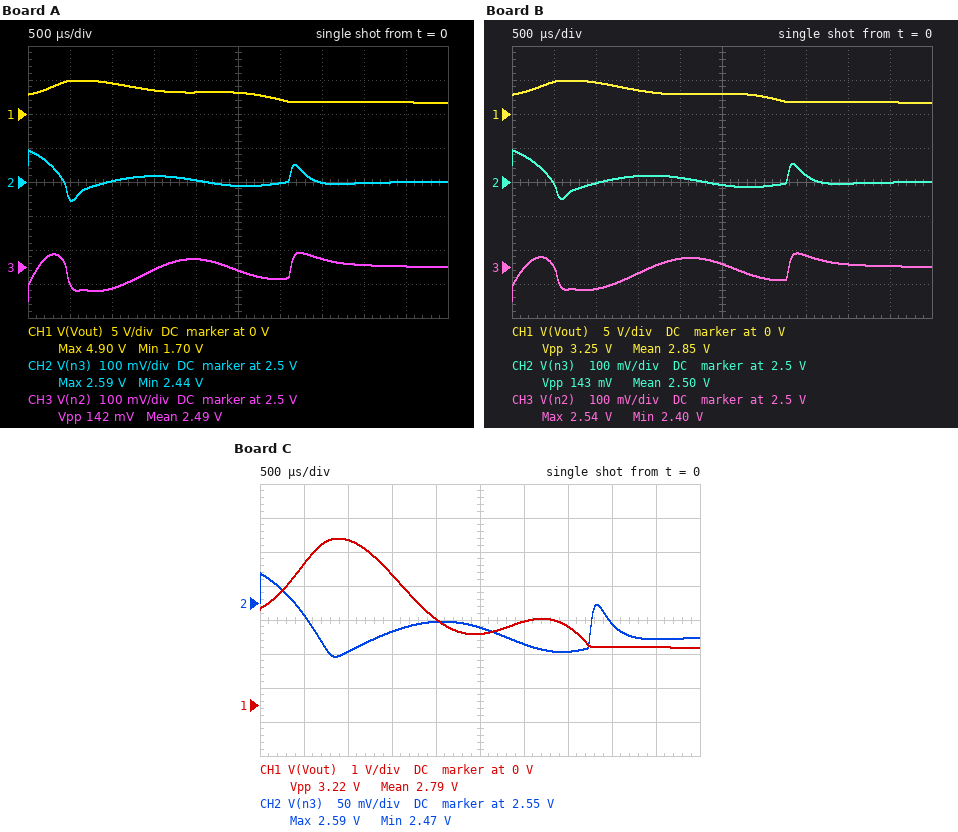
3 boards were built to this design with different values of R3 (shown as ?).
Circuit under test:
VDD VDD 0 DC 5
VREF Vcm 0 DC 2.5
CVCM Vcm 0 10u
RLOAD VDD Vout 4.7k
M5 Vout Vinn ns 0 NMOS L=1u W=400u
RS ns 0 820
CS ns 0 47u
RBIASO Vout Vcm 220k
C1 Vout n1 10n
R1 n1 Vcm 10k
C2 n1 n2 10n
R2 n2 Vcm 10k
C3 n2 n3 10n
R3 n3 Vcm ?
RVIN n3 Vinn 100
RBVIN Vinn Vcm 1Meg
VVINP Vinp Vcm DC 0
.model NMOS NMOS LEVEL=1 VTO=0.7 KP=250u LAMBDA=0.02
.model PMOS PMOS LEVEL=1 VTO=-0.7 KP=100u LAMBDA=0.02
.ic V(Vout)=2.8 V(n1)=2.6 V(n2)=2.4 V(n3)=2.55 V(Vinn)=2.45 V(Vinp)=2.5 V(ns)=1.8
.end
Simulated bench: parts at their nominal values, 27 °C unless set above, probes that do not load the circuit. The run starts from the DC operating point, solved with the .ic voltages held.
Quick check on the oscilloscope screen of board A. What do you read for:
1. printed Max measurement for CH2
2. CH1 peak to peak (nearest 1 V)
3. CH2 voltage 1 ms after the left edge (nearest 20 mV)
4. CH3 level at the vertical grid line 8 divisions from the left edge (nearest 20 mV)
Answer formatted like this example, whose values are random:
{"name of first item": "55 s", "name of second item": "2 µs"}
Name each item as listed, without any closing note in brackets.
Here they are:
{"printed Max measurement for CH2": "2.59 V", "CH1 peak to peak": "3 V", "CH2 voltage 1 ms after the left edge": "2.50 V", "CH3 level at the vertical grid line 8 divisions from the left edge": "2.50 V"}
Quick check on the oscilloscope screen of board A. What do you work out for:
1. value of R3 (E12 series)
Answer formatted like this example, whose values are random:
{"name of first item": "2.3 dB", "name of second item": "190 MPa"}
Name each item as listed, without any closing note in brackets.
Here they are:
{"value of R3": "15 kΩ"}
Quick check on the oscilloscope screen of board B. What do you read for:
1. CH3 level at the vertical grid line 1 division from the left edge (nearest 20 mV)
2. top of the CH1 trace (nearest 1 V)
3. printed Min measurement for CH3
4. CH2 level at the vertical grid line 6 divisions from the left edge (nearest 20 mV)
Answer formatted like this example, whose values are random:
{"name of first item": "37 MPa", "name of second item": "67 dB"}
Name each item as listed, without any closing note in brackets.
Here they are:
{"CH3 level at the vertical grid line 1 division from the left edge": "2.50 V", "top of the CH1 trace": "5 V", "printed Min measurement for CH3": "2.40 V", "CH2 level at the vertical grid line 6 divisions from the left edge": "2.48 V"}
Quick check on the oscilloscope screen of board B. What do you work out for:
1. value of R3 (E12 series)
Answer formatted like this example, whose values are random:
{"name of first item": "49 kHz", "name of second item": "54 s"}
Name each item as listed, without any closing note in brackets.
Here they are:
{"value of R3": "18 kΩ"}
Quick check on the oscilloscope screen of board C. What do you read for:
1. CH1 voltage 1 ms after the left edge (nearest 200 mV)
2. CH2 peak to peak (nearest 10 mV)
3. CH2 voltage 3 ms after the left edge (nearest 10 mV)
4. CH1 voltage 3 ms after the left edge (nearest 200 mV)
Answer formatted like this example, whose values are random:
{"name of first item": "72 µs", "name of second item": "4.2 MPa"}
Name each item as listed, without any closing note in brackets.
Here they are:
{"CH1 voltage 1 ms after the left edge": "4.8 V", "CH2 peak to peak": "120 mV", "CH2 voltage 3 ms after the left edge": "2.49 V", "CH1 voltage 3 ms after the left edge": "2.4 V"}
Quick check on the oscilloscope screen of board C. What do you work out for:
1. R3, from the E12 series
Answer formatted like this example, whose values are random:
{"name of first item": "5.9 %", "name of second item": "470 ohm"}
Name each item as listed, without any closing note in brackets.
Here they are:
{"R3, from the E12 series": "27 kΩ"}
